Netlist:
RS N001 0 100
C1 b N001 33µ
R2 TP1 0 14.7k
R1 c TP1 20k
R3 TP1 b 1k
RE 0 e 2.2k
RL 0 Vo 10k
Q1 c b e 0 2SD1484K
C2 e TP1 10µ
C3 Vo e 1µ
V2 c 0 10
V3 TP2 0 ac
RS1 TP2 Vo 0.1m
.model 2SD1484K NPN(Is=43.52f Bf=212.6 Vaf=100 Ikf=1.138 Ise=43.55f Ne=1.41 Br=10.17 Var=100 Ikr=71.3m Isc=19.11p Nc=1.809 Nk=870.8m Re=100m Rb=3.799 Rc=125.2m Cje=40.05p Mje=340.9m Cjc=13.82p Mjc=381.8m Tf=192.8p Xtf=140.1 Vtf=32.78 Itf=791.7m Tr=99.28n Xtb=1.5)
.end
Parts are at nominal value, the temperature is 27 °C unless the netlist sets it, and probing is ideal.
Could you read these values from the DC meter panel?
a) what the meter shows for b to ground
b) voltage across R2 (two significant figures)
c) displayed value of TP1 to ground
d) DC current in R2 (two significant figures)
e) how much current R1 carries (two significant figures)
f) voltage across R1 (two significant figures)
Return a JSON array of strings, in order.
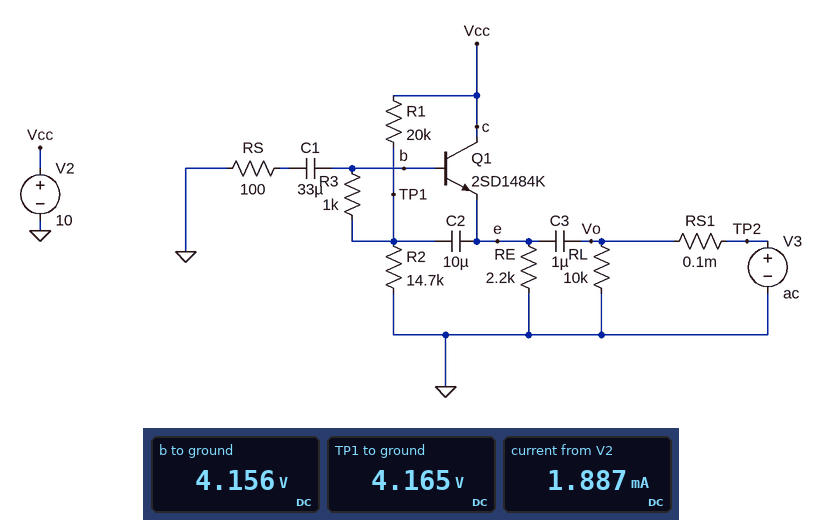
["4.156 V", "4.2 V", "4.165 V", "280 µA", "290 µA", "5.8 V"]
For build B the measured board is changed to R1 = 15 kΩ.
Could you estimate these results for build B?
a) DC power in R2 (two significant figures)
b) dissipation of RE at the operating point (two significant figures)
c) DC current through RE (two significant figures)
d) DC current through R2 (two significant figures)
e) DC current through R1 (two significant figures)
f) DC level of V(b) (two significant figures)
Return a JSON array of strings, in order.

["1.6 mW", "8.1 mW", "1.9 mA", "330 µA", "340 µA", "4.9 V"]
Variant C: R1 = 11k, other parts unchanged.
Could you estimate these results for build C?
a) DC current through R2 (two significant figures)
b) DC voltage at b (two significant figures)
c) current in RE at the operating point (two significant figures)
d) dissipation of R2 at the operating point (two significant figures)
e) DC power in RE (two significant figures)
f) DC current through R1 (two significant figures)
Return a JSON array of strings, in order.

["380 µA", "5.6 V", "2.3 mA", "2.2 mW", "11 mW", "400 µA"]
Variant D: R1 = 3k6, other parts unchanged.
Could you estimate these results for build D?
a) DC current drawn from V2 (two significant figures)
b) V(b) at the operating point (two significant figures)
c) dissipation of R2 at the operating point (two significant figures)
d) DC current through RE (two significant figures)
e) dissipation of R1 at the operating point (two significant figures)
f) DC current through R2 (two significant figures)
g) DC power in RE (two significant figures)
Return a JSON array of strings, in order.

["3.9 mA", "8.0 V", "4.3 mW", "3.3 mA", "1.1 mW", "540 µA", "24 mW"]
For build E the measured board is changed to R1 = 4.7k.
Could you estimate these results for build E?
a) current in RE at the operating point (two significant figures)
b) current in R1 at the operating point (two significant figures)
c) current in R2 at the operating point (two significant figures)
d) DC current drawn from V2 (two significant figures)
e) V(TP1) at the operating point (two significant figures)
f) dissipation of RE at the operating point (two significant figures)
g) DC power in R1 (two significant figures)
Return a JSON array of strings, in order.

["3.1 mA", "530 µA", "510 µA", "3.6 mA", "7.5 V", "21 mW", "1.3 mW"]
